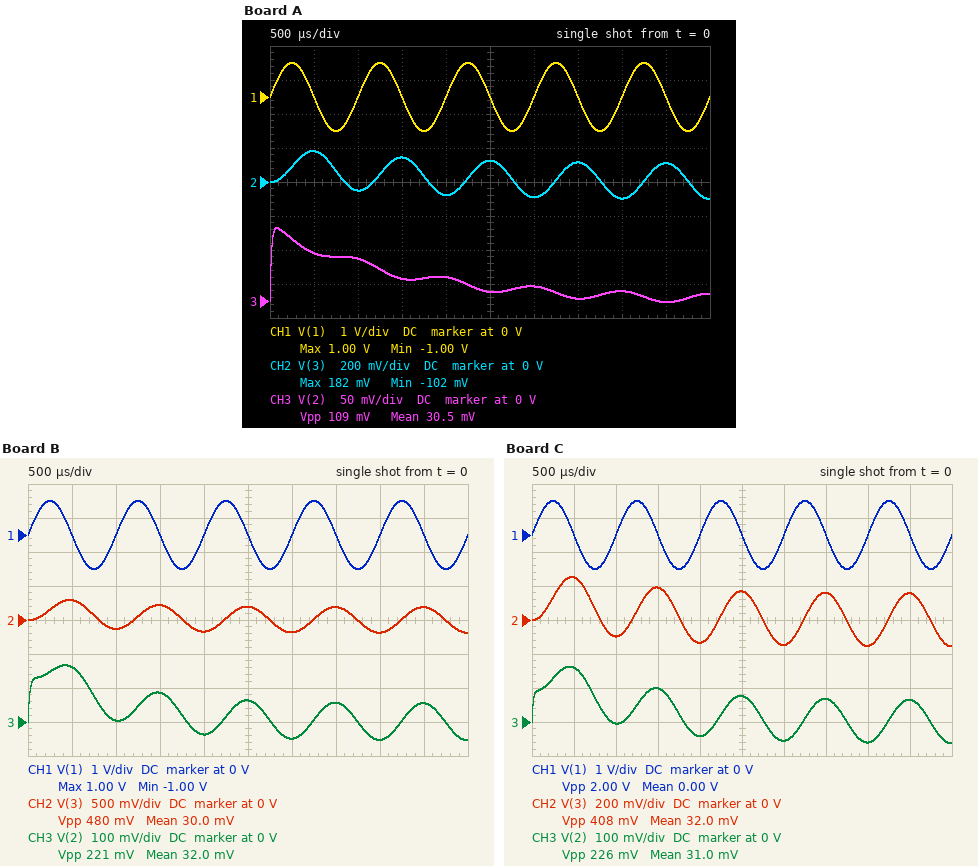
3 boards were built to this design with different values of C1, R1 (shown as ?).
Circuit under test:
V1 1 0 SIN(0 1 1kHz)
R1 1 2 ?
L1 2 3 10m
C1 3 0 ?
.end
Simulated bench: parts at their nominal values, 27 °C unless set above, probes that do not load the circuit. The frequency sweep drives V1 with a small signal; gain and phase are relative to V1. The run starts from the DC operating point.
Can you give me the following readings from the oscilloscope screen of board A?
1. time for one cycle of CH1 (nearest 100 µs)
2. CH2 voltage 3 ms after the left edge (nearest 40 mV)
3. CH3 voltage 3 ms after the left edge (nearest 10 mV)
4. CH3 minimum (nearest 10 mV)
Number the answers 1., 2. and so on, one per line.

1. 1.0 ms
2. -80 mV
3. 20 mV
4. 0 V
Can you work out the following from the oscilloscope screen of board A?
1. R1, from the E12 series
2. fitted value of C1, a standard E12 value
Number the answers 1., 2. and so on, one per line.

1. 560 Ω
2. 2.7 µF
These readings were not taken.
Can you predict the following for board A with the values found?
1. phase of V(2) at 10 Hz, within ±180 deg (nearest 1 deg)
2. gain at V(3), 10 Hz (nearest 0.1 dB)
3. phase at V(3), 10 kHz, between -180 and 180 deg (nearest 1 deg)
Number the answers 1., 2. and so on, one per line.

1. -5 deg
2. 0 dB
3. -138 deg
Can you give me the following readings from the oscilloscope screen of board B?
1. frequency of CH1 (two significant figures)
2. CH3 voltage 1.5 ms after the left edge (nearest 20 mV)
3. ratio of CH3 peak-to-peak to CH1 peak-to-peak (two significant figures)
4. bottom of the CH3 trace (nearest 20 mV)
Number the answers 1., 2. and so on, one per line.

1. 1.0 kHz
2. 80 mV
3. 0.11
4. -60 mV
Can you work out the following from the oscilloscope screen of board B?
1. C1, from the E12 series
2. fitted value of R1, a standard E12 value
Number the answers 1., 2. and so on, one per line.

1. 1.8 µF
2. 470 Ω
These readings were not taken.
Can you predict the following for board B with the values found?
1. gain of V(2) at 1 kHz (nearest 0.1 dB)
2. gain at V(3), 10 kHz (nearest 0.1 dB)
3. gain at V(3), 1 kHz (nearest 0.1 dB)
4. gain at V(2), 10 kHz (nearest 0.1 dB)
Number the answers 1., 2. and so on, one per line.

1. -25.3 dB
2. -38.9 dB
3. -14.5 dB
4. -2.0 dB
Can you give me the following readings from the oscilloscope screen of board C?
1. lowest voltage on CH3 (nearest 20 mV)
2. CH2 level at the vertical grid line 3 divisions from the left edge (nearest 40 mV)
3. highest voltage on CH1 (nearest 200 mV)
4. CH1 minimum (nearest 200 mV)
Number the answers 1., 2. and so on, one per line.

1. -60 mV
2. 200 mV
3. 1.0 V
4. -1.0 V
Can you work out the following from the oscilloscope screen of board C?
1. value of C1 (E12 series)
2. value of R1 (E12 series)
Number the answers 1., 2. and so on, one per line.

1. 1.5 µF
2. 680 Ω
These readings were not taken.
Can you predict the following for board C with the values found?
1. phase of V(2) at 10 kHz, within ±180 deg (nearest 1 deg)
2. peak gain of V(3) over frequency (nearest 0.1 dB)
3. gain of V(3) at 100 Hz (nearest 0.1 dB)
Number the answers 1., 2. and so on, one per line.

1. 48 deg
2. 0 dB
3. -1.5 dB
